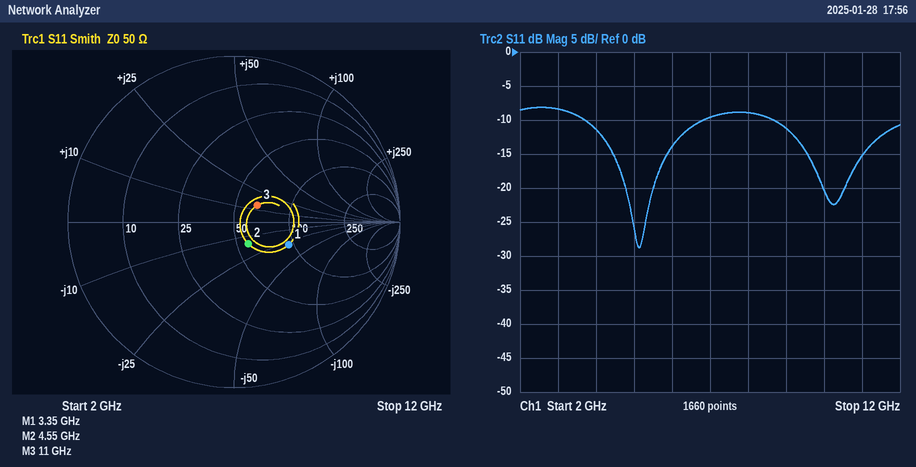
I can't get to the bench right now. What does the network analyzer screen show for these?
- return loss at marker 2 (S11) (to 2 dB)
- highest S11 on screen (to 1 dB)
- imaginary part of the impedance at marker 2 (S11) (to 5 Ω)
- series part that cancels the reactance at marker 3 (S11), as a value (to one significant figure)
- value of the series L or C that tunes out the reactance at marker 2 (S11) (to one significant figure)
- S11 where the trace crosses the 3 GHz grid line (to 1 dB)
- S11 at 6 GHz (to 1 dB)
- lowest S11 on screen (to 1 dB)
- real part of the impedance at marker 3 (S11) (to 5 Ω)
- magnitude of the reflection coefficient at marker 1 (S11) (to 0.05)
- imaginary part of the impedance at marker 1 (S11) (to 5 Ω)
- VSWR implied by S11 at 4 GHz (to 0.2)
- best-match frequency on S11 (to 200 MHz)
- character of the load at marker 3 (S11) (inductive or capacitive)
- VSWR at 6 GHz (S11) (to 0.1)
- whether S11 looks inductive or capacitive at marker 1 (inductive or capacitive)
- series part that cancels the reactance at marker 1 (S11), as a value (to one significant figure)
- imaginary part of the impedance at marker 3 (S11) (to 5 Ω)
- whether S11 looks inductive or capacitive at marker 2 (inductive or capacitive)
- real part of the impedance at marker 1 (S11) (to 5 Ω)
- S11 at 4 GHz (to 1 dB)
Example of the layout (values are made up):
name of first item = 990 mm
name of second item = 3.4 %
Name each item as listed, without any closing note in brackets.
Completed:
return loss at marker 2 (S11) = 16 dB
highest S11 on screen = -8 dB
imaginary part of the impedance at marker 2 (S11) = -15 Ω
series part that cancels the reactance at marker 3 (S11), as a value = 1 pF
value of the series L or C that tunes out the reactance at marker 2 (S11) = 500 pH
S11 where the trace crosses the 3 GHz grid line = -8 dB
S11 at 6 GHz = -14 dB
lowest S11 on screen = -29 dB
real part of the impedance at marker 3 (S11) = 65 Ω
magnitude of the reflection coefficient at marker 1 (S11) = 0.35
imaginary part of the impedance at marker 1 (S11) = -30 Ω
VSWR implied by S11 at 4 GHz = 1.8
best-match frequency on S11 = 5.2 GHz
character of the load at marker 3 (S11) = inductive
VSWR at 6 GHz (S11) = 1.5
whether S11 looks inductive or capacitive at marker 1 = capacitive
series part that cancels the reactance at marker 1 (S11), as a value = 1 nH
imaginary part of the impedance at marker 3 (S11) = +15 Ω
whether S11 looks inductive or capacitive at marker 2 = capacitive
real part of the impedance at marker 1 (S11) = 95 Ω
S11 at 4 GHz = -11 dB
